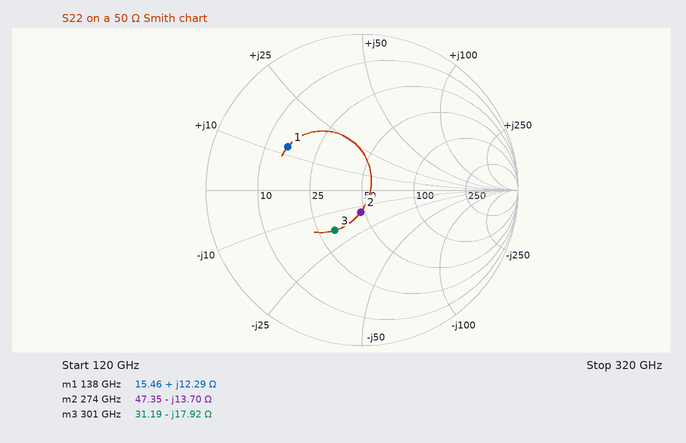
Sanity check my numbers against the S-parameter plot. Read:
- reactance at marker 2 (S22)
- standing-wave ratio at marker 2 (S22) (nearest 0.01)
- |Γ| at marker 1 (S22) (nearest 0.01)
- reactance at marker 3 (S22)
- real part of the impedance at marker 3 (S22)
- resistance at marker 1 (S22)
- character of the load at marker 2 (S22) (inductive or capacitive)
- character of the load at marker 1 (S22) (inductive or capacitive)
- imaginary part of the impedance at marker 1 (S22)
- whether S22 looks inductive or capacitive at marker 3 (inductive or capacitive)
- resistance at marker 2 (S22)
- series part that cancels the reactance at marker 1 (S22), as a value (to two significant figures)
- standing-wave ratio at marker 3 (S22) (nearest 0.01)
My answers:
-13.70 Ω
1.33
0.55
-17.92 Ω
31.19 Ω
15.46 Ω
capacitive
inductive
+12.29 Ω
capacitive
47.35 Ω
94 fF
1.91
